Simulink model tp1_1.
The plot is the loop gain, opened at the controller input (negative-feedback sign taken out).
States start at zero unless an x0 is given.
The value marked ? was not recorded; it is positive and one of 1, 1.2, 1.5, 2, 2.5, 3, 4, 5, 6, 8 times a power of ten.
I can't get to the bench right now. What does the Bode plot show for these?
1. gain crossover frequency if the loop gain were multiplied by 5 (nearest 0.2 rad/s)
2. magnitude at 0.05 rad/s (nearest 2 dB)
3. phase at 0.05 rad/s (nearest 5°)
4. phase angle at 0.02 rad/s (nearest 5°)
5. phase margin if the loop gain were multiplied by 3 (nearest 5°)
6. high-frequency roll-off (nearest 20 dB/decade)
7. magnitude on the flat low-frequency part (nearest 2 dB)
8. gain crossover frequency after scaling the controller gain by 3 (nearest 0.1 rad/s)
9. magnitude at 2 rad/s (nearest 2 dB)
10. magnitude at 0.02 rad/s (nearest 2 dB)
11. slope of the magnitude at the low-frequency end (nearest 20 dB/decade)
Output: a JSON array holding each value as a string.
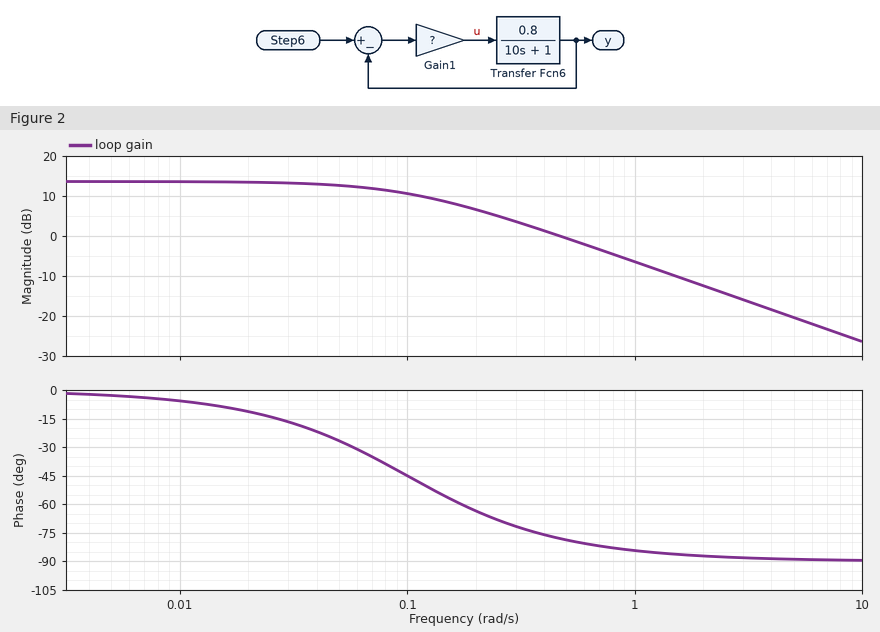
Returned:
["2.4 rad/s", "12 dB", "-25°", "-10°", "95°", "-20 dB/decade", "14 dB", "1.4 rad/s", "-12 dB", "14 dB", "0 dB/decade"]
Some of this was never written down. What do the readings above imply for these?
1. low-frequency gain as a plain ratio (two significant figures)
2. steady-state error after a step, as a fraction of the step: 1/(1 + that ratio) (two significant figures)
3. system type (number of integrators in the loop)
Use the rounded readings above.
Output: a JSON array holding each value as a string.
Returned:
["5.0", "0.17", "0"]
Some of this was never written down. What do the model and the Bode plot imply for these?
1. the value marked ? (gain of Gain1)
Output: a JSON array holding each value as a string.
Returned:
["6"]
